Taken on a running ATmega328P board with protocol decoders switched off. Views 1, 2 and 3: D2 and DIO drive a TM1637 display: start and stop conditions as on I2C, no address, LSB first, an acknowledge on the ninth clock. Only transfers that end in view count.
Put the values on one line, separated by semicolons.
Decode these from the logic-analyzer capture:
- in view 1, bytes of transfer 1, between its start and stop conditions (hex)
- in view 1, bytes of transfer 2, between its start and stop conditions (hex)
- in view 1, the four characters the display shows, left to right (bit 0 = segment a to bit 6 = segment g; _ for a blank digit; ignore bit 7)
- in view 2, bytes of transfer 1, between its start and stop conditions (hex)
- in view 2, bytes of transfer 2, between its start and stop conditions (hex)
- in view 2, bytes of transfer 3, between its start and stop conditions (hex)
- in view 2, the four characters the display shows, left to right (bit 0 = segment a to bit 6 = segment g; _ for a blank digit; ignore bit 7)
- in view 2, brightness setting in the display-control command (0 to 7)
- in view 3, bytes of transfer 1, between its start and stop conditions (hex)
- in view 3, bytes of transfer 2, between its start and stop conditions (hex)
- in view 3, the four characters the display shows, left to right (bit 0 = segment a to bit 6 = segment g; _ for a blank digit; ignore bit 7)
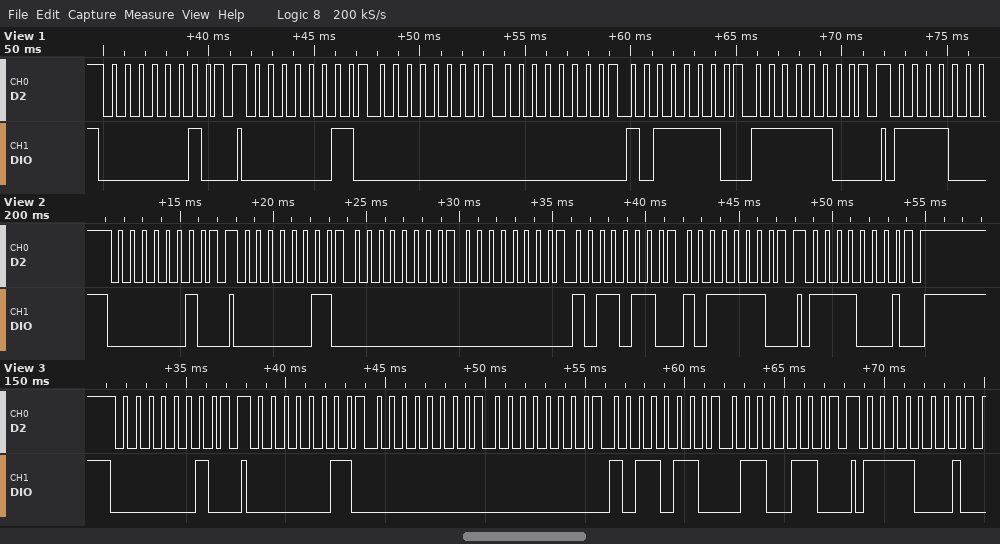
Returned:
40; C0 00 00 7D 3F; __60; 40; C0 00 00 6D 7D; 8F; __56; 7; 40; C0 00 00 6D 66; __54
